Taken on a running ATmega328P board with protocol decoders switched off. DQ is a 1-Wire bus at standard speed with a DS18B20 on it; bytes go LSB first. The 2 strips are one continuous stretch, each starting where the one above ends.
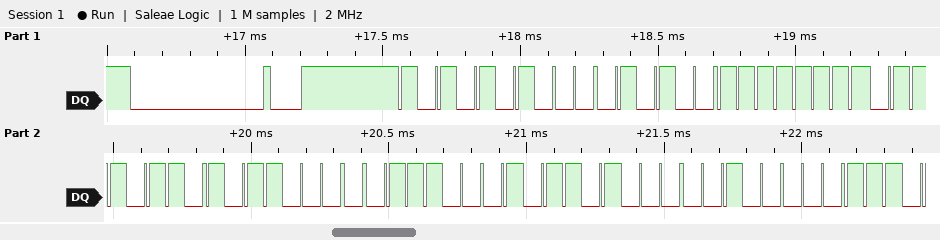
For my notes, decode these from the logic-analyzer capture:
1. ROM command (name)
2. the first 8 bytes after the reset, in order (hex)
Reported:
Match ROM
55 28 FF 6E 0D 8E 16 04
